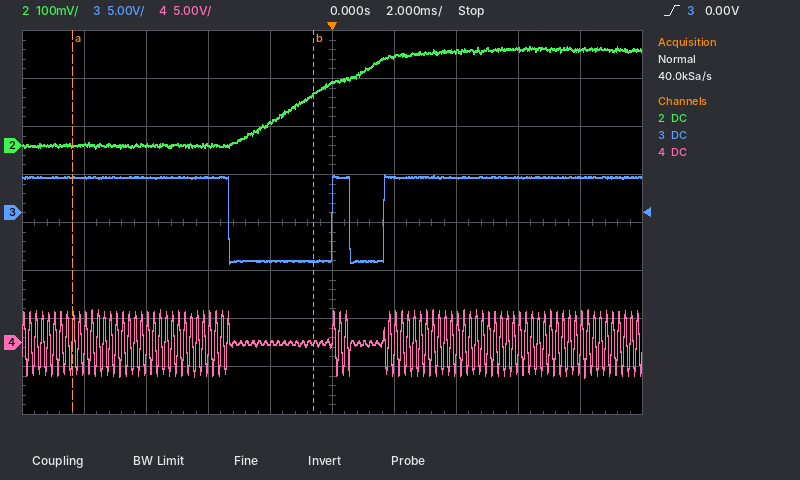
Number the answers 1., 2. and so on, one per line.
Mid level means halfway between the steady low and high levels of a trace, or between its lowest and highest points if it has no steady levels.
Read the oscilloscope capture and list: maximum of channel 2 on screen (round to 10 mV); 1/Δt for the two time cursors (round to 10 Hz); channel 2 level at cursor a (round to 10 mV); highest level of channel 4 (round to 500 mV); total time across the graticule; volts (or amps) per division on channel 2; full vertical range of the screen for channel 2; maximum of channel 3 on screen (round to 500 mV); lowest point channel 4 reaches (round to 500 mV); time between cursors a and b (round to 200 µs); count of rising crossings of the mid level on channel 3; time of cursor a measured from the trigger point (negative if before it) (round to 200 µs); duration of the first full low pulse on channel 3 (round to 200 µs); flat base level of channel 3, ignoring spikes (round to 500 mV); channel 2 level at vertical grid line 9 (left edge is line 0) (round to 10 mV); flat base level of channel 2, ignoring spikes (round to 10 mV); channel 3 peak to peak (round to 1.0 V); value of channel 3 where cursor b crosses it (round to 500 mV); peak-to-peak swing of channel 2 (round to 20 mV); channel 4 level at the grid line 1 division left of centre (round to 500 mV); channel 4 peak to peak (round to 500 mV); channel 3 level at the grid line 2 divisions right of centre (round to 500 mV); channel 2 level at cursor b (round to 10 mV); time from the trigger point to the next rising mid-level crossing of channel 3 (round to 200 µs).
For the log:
1. 210 mV
2. 130 Hz
3. 0 mV
4. 3.5 V
5. 20 ms
6. 100 mV
7. 800 mV
8. 4.0 V
9. -3.5 V
10. 7.8 ms
11. 2
12. -8.4 ms
13. 3.4 ms
14. -5.0 V
15. 200 mV
16. 0 mV
17. 9.0 V
18. -5.0 V
19. 220 mV
20. 0.0 V
21. 7.0 V
22. 3.5 V
23. 110 mV
24. 1.6 ms
